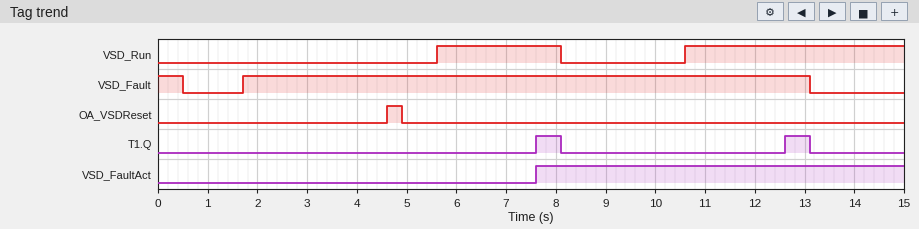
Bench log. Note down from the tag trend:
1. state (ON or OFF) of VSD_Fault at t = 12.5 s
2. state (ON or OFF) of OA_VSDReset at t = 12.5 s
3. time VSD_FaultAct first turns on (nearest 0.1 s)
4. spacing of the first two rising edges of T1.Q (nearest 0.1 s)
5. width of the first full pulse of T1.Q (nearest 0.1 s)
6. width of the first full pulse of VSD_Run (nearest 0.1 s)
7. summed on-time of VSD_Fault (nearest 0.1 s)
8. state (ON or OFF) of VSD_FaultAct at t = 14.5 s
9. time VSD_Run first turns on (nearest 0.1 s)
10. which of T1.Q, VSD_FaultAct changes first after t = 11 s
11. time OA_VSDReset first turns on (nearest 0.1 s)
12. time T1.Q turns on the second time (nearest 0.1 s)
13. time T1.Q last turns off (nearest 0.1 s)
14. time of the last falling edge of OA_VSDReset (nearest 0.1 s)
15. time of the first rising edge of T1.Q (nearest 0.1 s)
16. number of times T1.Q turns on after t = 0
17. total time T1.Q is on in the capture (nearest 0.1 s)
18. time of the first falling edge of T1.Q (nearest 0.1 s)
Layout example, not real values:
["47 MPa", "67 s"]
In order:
["ON", "OFF", "7.6 s", "5.0 s", "0.5 s", "2.5 s", "11.9 s", "ON", "5.6 s", "T1.Q", "4.6 s", "12.6 s", "13.1 s", "4.9 s", "7.6 s", "2", "1.0 s", "8.1 s"]
